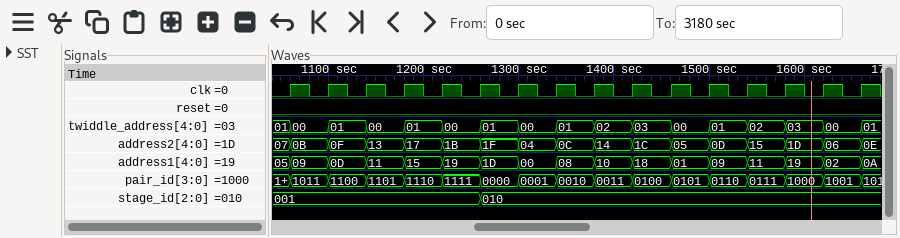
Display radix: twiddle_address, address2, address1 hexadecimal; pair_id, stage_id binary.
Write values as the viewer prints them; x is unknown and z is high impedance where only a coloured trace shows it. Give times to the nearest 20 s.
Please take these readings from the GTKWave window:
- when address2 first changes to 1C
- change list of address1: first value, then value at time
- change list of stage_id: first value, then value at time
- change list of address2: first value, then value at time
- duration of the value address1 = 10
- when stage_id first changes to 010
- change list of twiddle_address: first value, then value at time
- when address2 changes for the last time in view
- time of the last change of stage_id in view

1420 s
05, 09 at 1060 s, 0D at 1100 s, 11 at 1140 s, 15 at 1180 s, 19 at 1220 s, 1D at 1260 s, 00 at 1300 s, 08 at 1340 s, 10 at 1380 s, 18 at 1420 s, 01 at 1460 s, 09 at 1500 s, 11 at 1540 s, 19 at 1580 s, 02 at 1620 s, 0A at 1660 s
001, 010 at 1260 s
07, 0B at 1060 s, 0F at 1100 s, 13 at 1140 s, 17 at 1180 s, 1B at 1220 s, 1F at 1260 s, 04 at 1300 s, 0C at 1340 s, 14 at 1380 s, 1C at 1420 s, 05 at 1460 s, 0D at 1500 s, 15 at 1540 s, 1D at 1580 s, 06 at 1620 s, 0E at 1660 s
40 s
1260 s
01, 00 at 1060 s, 01 at 1100 s, 00 at 1140 s, 01 at 1180 s, 00 at 1220 s, 01 at 1260 s, 00 at 1300 s, 01 at 1340 s, 02 at 1380 s, 03 at 1420 s, 00 at 1460 s, 01 at 1500 s, 02 at 1540 s, 03 at 1580 s, 00 at 1620 s, 01 at 1660 s
1660 s
1260 s
